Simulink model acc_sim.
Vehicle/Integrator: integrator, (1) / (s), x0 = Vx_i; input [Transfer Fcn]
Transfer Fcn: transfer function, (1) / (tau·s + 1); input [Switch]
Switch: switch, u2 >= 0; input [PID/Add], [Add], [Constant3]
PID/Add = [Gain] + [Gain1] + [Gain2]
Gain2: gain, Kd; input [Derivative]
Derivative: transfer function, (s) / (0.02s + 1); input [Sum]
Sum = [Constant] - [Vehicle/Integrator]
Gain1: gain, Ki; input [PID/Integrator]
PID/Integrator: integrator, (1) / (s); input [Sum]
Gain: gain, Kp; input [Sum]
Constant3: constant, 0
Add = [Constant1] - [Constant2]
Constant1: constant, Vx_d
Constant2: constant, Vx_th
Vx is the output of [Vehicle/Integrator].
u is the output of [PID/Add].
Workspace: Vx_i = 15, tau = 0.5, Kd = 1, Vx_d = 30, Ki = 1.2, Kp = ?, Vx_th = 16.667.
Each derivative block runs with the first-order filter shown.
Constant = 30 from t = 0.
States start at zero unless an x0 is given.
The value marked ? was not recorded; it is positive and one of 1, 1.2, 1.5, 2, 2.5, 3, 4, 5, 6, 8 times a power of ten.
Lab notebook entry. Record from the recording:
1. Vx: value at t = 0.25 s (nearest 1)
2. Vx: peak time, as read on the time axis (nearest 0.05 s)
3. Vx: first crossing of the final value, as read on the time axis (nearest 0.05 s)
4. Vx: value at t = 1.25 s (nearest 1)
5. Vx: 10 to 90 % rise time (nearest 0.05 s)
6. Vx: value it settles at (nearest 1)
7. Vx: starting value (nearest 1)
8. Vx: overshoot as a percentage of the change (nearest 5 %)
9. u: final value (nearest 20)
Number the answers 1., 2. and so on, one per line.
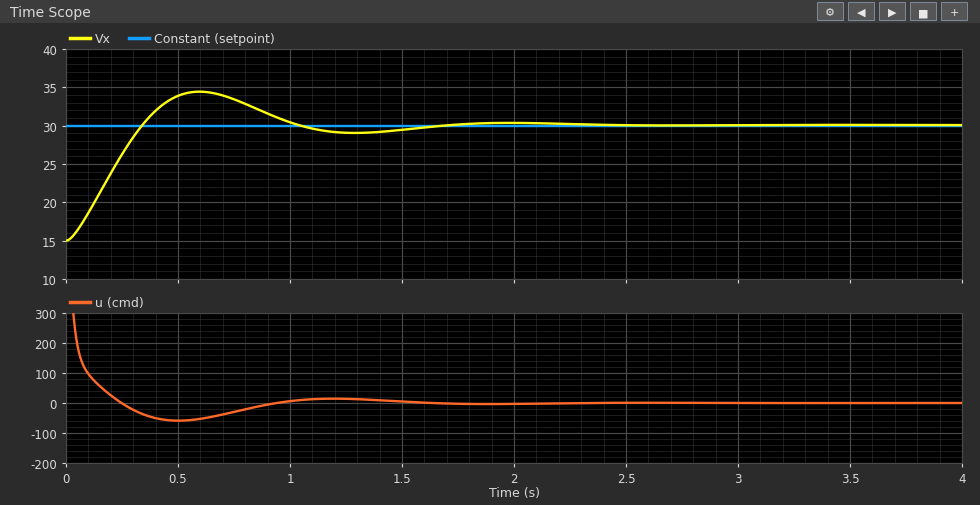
1. 26
2. 0.60 s
3. 0.35 s
4. 29
5. 0.25 s
6. 30
7. 15
8. 30 %
9. 0
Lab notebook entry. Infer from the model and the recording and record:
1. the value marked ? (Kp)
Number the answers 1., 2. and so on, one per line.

1. 12
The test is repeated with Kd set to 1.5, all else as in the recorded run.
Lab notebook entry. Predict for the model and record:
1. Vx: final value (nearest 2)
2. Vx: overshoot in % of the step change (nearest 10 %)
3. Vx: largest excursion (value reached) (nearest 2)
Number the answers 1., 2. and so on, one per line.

1. 30
2. 20 %
3. 34
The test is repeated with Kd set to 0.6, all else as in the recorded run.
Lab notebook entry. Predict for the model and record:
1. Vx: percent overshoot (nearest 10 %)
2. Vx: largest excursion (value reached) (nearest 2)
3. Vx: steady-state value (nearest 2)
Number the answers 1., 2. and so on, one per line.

1. 40 %
2. 36
3. 30
